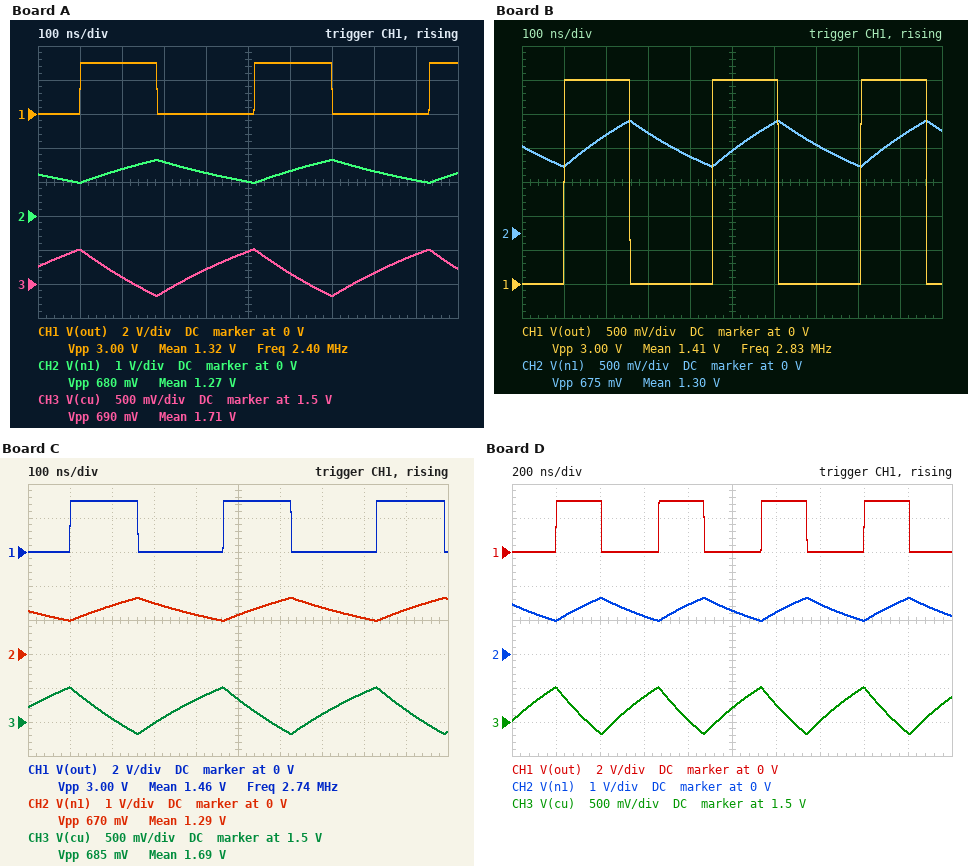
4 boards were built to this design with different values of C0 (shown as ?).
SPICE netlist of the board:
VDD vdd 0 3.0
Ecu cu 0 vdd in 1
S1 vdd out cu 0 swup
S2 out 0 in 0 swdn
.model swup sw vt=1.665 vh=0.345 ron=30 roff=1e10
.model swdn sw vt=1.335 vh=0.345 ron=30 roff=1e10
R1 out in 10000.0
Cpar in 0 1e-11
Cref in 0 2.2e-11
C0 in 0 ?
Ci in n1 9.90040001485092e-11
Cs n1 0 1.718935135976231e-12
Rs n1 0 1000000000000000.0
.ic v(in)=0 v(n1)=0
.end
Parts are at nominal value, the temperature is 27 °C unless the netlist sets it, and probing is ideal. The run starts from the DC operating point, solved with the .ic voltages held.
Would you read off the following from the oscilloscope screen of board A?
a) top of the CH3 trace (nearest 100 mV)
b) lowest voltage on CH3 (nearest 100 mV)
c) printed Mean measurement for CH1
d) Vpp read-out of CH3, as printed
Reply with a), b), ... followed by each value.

a) 2.0 V
b) 1.3 V
c) 1.32 V
d) 690 mV
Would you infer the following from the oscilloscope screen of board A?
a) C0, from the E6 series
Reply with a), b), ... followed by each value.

a) 10 pF
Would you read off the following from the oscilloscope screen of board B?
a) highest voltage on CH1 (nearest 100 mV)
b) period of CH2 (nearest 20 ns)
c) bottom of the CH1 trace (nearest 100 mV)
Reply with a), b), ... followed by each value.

a) 3.0 V
b) 360 ns
c) 0 V
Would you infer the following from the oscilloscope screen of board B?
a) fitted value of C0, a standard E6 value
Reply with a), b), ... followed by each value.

a) 3.3 pF
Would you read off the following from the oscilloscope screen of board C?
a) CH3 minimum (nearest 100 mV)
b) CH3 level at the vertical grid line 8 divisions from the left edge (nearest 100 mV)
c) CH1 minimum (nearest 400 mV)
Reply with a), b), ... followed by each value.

a) 1.3 V
b) 1.9 V
c) 0 V
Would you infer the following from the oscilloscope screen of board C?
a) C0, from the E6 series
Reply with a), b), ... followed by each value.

a) 4.7 pF
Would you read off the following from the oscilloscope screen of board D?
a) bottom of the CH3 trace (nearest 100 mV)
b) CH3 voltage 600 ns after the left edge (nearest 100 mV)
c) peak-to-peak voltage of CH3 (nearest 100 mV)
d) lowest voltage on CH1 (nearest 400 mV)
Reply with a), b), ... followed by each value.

a) 1.3 V
b) 1.9 V
c) 700 mV
d) 0 V
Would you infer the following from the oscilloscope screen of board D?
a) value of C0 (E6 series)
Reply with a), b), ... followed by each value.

a) 15 pF
